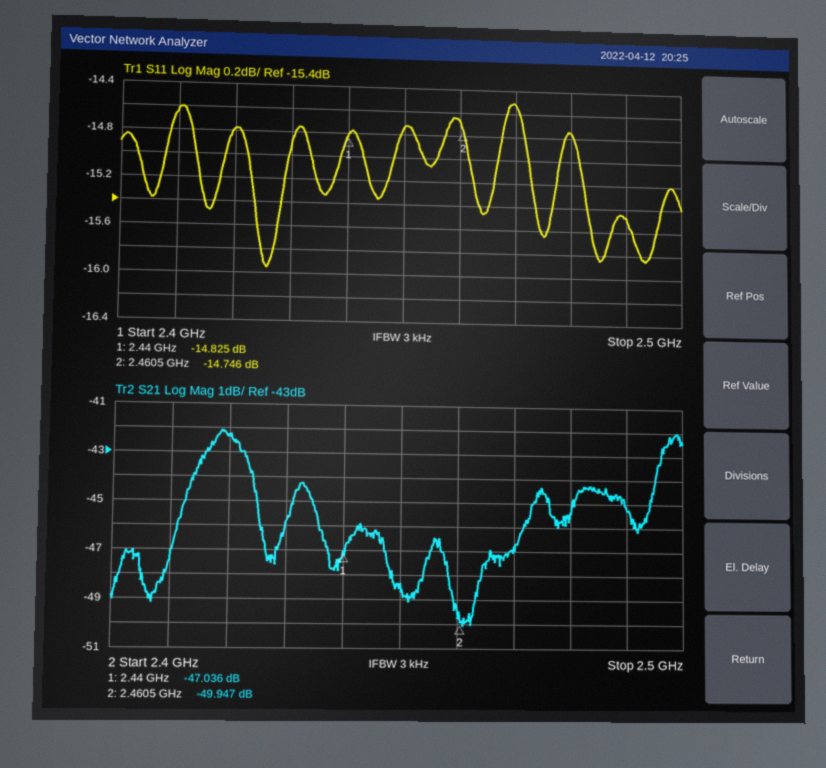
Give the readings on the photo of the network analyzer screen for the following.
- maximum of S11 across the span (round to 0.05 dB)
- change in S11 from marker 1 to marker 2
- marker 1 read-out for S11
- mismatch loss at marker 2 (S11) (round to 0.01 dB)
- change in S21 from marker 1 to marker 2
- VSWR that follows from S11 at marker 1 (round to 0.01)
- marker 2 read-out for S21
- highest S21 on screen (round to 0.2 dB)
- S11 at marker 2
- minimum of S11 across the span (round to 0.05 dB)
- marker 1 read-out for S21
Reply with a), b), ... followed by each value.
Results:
a) -14.50 dB
b) 0.079 dB
c) -14.825 dB
d) 0.15 dB
e) -2.911 dB
f) 1.44
g) -49.947 dB
h) -42.0 dB
i) -14.746 dB
j) -15.95 dB
k) -47.036 dB
